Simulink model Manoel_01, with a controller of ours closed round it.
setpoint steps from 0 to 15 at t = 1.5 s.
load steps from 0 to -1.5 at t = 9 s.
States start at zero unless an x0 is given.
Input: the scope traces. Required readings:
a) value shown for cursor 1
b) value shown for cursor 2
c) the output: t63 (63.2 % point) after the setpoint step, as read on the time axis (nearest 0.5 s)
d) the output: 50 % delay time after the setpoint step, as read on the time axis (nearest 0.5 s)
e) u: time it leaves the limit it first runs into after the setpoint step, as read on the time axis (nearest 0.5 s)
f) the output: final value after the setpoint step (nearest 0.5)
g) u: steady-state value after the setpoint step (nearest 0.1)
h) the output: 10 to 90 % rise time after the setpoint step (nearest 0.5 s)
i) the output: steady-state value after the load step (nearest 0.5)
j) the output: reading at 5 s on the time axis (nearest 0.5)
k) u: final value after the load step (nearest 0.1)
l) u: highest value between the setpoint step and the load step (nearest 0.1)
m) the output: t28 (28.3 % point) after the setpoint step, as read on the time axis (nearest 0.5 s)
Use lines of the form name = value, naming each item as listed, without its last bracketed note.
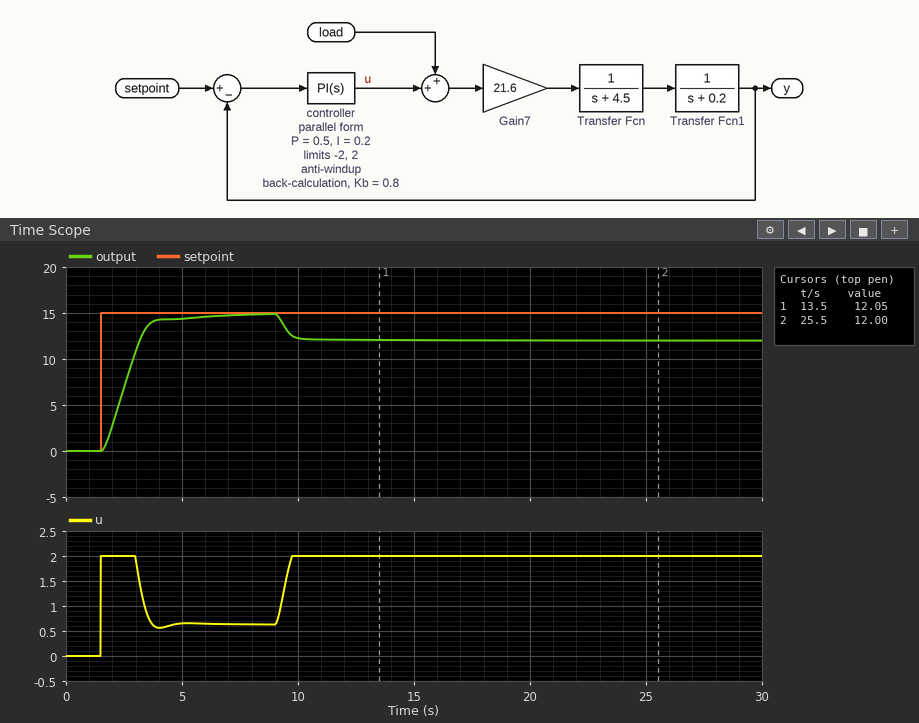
value shown for cursor 1 = 12.05
value shown for cursor 2 = 12.00
the output: t63 (63.2 % point) after the setpoint step, as read on the time axis = 3.0 s
the output: 50 % delay time after the setpoint step, as read on the time axis = 2.5 s
u: time it leaves the limit it first runs into after the setpoint step, as read on the time axis = 3.0 s
the output: final value after the setpoint step = 15.0
u: steady-state value after the setpoint step = 0.6
the output: 10 to 90 % rise time after the setpoint step = 1.5 s
the output: steady-state value after the load step = 12.0
the output: reading at 5 s on the time axis = 14.5
u: final value after the load step = 2.0
u: highest value between the setpoint step and the load step = 2.0
the output: t28 (28.3 % point) after the setpoint step, as read on the time axis = 2.0 s
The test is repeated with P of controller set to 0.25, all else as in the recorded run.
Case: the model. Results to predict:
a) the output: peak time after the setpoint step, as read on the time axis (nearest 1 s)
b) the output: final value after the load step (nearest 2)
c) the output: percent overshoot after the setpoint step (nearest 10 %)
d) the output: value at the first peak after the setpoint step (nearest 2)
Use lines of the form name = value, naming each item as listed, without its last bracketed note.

the output: peak time after the setpoint step, as read on the time axis = 5 s
the output: final value after the load step = 12
the output: percent overshoot after the setpoint step = 20 %
the output: value at the first peak after the setpoint step = 18
